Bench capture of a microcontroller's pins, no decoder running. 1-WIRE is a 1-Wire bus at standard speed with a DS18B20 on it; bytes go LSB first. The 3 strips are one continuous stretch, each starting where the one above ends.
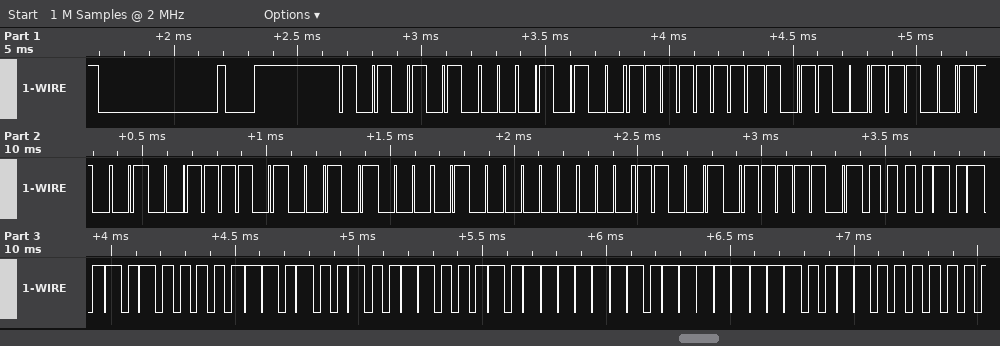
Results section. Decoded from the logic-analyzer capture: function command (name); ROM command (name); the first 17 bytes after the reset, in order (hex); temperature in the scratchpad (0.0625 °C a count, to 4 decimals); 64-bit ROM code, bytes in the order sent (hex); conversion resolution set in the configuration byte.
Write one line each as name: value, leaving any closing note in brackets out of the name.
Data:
function command: Read Scratchpad
ROM command: Match ROM
the first 17 bytes after the reset, in order: 55 28 FF CD 99 BC 14 02 98 BE 50 05 4B 46 7F FF 0C
temperature in the scratchpad: 85.0000 °C
64-bit ROM code, bytes in the order sent: 28 FF CD 99 BC 14 02 98
conversion resolution set in the configuration byte: 12 bits
